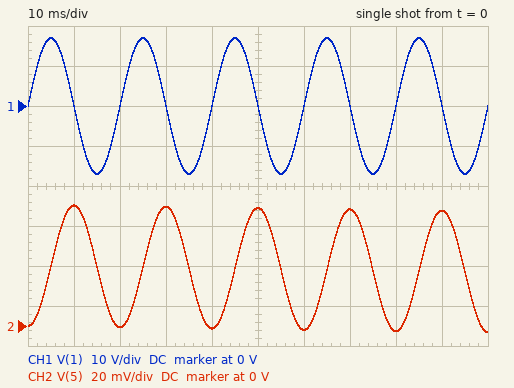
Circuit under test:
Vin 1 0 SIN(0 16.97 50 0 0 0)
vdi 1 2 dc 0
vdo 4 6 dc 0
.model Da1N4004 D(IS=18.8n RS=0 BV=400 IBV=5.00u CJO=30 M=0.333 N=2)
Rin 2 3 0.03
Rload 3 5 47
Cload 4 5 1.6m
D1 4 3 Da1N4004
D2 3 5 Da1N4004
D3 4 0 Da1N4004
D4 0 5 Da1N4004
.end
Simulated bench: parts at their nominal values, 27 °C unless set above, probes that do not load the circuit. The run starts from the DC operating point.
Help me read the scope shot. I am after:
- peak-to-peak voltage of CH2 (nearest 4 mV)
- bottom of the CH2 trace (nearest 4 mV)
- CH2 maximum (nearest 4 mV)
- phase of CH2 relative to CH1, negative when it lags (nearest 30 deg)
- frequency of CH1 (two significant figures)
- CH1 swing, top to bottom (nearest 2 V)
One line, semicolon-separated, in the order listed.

64 mV; -4 mV; 60 mV; -90 deg; 50 Hz; 34 V
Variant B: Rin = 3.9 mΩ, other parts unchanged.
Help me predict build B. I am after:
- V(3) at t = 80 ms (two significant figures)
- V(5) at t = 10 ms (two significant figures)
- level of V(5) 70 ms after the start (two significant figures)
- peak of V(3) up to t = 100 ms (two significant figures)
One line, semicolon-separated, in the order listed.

-230 mV; 470 mV; 380 mV; 880 mV
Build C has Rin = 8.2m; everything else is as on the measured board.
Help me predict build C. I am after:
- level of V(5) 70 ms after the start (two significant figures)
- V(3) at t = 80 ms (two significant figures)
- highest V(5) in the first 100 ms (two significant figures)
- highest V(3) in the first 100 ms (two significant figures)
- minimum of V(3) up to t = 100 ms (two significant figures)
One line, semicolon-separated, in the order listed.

200 mV; -61 mV; 220 mV; 430 mV; -73 mV
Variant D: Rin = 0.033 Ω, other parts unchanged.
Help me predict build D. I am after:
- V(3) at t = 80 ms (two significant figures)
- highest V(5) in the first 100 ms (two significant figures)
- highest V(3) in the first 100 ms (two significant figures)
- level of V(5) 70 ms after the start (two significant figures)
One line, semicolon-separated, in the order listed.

-4.2 mV; 55 mV; 110 mV; 53 mV
